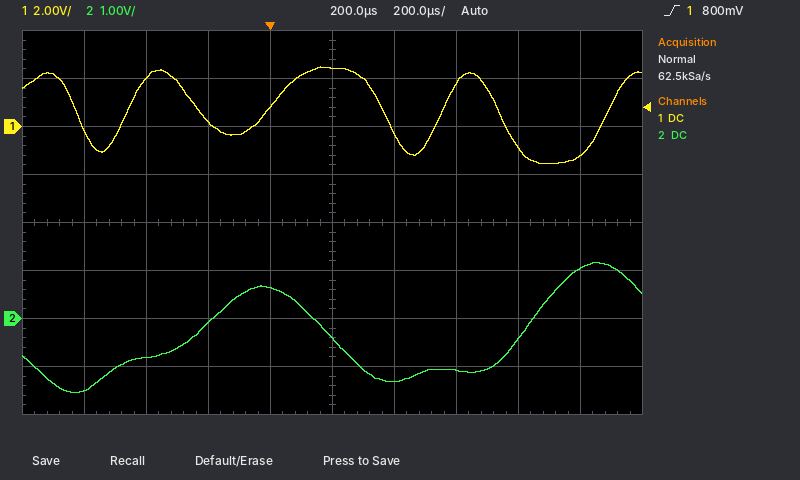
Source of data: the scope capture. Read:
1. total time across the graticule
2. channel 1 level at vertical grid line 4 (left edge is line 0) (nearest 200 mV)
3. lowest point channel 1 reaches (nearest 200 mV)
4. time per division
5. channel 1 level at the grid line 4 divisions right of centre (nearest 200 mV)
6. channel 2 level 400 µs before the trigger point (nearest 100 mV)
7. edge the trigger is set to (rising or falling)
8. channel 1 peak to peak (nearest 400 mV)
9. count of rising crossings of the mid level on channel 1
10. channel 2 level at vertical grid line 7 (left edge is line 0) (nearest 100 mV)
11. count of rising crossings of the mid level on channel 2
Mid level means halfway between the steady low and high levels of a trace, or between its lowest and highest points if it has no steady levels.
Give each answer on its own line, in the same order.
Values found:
2 ms
800 mV
-1.6 V
200 µs
-1.2 V
-800 mV
rising
4.0 V
4
-1.1 V
2
